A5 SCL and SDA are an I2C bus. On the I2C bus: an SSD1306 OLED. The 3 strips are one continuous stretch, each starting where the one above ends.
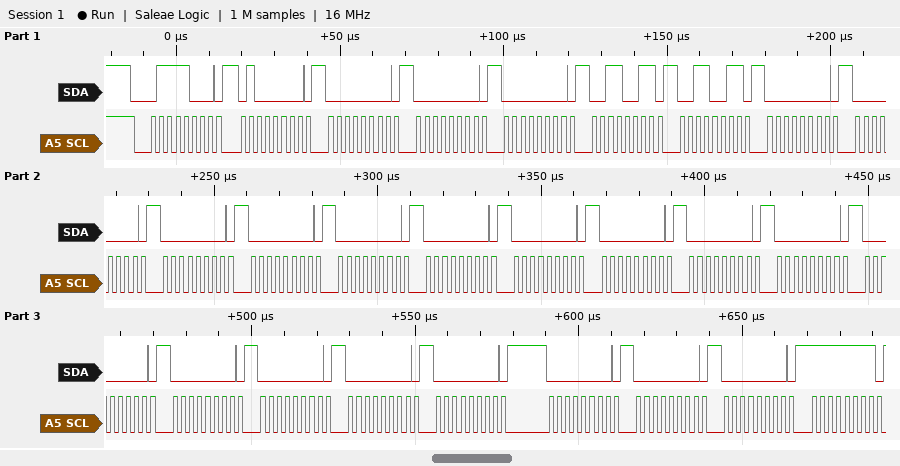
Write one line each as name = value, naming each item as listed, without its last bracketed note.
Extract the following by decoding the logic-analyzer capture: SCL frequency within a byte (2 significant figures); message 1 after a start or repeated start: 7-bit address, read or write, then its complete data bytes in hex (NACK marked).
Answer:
SCL frequency within a byte = 400 kHz
message 1 after a start or repeated start: 7-bit address, read or write, then its complete data bytes in hex = 0x3C write: 40 00 00 00 33 33 00 00 00 00 00 00 00 00 00 00 00 00 00 00 00 00 00 00 FF
